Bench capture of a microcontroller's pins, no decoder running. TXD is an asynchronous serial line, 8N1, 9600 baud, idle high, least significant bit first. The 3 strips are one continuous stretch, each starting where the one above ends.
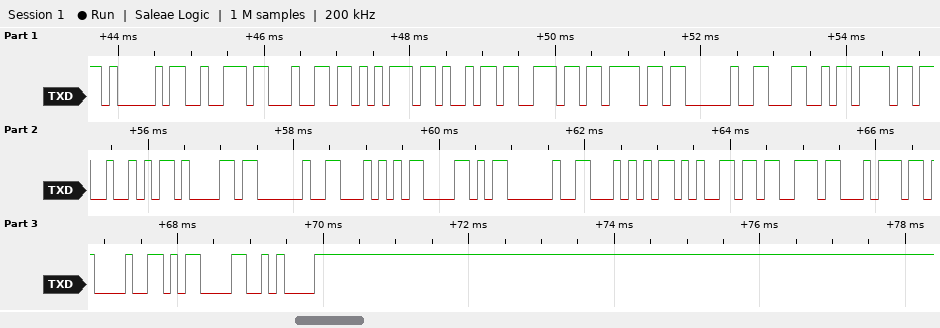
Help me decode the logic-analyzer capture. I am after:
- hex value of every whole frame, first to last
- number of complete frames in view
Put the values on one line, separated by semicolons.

41 72 64 75 69 6E 6F 20 4C 6F 52 61 20 54 58 20 54 65 73 74 21 0D 0A; 23
